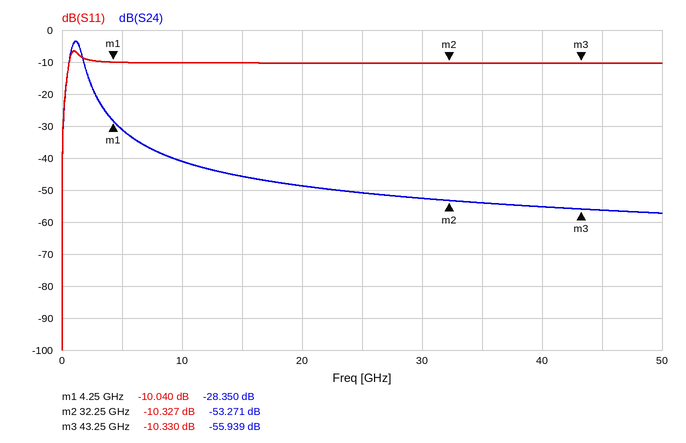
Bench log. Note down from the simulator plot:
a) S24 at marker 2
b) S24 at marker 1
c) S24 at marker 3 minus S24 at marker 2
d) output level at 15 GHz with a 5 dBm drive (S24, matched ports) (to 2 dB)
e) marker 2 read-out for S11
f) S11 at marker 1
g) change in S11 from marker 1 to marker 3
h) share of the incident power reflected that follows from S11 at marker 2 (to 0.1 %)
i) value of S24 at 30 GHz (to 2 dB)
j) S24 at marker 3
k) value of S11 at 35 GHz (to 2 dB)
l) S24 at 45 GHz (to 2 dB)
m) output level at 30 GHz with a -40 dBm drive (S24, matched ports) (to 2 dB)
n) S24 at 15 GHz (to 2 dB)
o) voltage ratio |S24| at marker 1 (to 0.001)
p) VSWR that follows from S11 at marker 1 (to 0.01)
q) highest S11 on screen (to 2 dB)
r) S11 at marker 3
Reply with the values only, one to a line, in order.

-53.271 dB
-28.350 dB
-2.668 dB
-40 dBm
-10.327 dB
-10.040 dB
-0.290 dB
9.3 %
-52 dB
-55.939 dB
-10 dB
-56 dB
-92 dBm
-46 dB
0.038
1.92
-6 dB
-10.330 dB
